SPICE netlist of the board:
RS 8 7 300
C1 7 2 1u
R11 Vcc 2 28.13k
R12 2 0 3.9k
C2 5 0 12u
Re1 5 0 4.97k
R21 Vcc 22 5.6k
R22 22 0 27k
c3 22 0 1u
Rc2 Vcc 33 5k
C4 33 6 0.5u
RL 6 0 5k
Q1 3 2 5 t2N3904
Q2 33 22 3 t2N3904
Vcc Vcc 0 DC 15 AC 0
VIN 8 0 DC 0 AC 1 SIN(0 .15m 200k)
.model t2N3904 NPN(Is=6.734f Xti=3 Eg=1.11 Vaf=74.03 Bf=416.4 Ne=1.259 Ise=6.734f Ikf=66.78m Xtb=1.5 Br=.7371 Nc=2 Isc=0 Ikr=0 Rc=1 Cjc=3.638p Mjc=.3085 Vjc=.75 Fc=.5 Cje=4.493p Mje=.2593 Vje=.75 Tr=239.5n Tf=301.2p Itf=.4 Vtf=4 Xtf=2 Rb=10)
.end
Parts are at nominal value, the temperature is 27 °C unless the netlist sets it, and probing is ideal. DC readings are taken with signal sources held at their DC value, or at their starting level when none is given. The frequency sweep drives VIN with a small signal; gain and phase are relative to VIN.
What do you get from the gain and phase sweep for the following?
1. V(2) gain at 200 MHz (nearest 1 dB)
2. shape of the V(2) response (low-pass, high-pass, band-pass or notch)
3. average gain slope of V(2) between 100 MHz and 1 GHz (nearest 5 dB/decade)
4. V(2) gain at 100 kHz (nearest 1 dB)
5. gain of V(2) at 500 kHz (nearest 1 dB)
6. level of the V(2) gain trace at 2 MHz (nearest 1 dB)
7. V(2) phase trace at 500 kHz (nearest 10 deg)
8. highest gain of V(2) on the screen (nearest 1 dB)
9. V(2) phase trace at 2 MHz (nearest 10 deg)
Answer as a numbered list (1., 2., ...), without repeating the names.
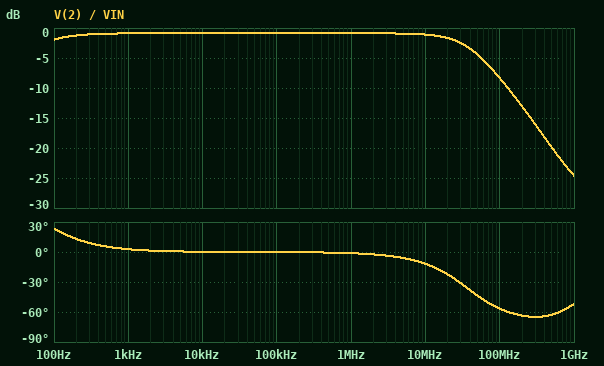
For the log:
1. -13 dB
2. low-pass
3. -15 dB/decade
4. -1 dB
5. -1 dB
6. -1 dB
7. 0 deg
8. -1 dB
9. 0 deg
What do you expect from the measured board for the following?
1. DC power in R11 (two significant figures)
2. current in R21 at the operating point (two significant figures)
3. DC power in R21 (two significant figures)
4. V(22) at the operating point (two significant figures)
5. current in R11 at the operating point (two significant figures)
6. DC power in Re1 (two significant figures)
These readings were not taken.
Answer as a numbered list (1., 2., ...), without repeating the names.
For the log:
1. 6.2 mW
2. 460 µA
3. 1.2 mW
4. 12 V
5. 470 µA
6. 290 µW
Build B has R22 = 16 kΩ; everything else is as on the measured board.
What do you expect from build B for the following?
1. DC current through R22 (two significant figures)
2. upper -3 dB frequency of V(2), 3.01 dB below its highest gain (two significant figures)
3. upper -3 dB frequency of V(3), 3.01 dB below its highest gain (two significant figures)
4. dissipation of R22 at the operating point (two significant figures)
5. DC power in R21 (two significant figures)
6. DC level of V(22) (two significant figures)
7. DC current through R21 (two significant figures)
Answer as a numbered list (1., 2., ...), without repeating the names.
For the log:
1. 690 µA
2. 44 MHz
3. 45 MHz
4. 7.7 mW
5. 2.7 mW
6. 11 V
7. 700 µA
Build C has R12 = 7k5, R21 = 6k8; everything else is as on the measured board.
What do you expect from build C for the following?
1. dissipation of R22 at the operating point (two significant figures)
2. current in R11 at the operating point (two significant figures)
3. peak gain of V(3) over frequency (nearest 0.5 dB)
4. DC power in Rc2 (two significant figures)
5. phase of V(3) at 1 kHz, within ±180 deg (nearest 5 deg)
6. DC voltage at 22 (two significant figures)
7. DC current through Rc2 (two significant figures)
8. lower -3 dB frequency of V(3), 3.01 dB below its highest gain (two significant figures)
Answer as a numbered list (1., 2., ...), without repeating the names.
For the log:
1. 5.3 mW
2. 420 µA
3. -0.5 dB
4. 1.2 mW
5. -165 deg
6. 12 V
7. 490 µA
8. 260 Hz
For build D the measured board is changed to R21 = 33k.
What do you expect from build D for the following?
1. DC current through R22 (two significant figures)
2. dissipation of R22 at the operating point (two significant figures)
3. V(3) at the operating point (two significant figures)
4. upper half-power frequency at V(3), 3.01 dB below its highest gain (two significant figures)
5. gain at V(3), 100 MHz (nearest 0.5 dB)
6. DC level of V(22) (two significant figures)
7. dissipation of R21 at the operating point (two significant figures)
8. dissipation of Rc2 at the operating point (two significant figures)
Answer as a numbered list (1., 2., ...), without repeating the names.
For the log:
1. 250 µA
2. 1.7 mW
3. 6.1 V
4. 42 MHz
5. -10.0 dB
6. 6.7 V
7. 2.1 mW
8. 280 µW
